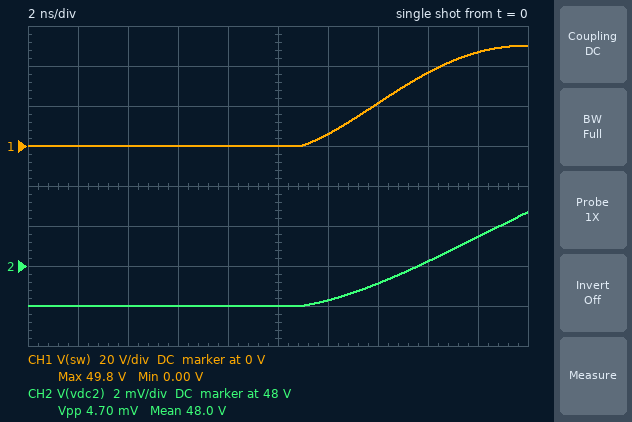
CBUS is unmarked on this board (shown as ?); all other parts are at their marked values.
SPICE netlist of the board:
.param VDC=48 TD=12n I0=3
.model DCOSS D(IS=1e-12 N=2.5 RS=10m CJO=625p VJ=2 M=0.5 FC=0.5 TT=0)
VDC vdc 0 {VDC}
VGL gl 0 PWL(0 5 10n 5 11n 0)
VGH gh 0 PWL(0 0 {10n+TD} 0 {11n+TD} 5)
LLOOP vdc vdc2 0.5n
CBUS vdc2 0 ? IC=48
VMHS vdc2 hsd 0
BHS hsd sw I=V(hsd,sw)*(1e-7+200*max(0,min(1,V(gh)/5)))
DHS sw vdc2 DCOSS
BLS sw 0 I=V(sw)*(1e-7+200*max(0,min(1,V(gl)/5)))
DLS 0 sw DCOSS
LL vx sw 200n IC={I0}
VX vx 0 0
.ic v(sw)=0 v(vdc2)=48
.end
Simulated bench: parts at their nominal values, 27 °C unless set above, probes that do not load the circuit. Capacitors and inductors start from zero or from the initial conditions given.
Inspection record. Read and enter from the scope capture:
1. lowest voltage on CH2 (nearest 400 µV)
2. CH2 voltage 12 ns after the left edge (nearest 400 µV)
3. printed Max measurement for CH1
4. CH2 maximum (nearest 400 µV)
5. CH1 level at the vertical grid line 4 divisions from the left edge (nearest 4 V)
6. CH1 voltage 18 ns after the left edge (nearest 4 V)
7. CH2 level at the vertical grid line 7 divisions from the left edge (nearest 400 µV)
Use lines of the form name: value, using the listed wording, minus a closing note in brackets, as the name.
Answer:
lowest voltage on CH2: 48.0000 V
CH2 voltage 12 ns after the left edge: 48.0004 V
printed Max measurement for CH1: 49.8 V
CH2 maximum: 48.0048 V
CH1 level at the vertical grid line 4 divisions from the left edge: 0 V
CH1 voltage 18 ns after the left edge: 48 V
CH2 level at the vertical grid line 7 divisions from the left edge: 48.0012 V
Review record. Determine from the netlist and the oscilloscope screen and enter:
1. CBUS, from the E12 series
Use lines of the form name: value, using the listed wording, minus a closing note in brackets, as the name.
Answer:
CBUS, from the E12 series: 2.7 µF
